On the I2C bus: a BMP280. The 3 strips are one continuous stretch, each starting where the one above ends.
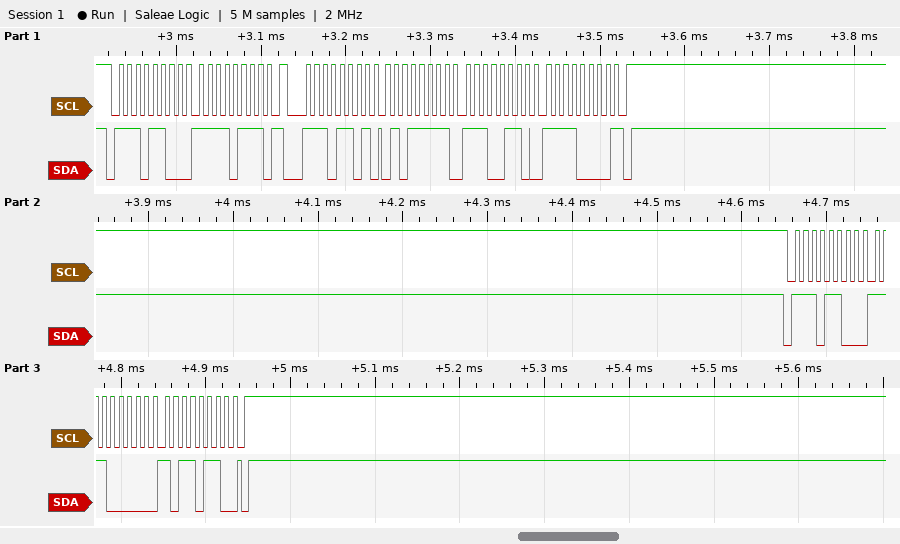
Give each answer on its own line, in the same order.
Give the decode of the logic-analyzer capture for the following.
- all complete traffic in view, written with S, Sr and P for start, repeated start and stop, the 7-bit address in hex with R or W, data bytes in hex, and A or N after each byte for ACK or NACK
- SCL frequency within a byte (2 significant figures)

S 76W A F7 A Sr 76R A 5F A E6 A F0 N P S 76W A E0 A B6 A P
100 kHz
